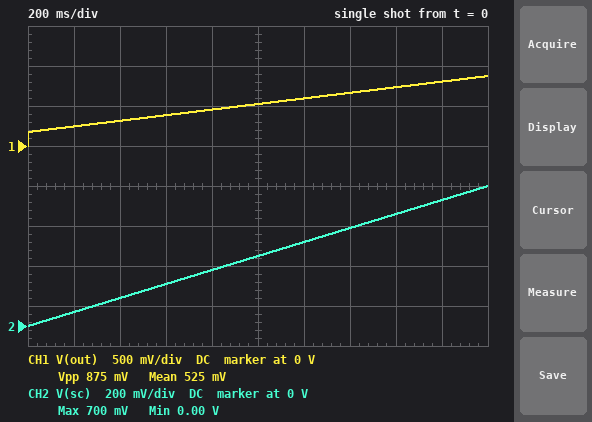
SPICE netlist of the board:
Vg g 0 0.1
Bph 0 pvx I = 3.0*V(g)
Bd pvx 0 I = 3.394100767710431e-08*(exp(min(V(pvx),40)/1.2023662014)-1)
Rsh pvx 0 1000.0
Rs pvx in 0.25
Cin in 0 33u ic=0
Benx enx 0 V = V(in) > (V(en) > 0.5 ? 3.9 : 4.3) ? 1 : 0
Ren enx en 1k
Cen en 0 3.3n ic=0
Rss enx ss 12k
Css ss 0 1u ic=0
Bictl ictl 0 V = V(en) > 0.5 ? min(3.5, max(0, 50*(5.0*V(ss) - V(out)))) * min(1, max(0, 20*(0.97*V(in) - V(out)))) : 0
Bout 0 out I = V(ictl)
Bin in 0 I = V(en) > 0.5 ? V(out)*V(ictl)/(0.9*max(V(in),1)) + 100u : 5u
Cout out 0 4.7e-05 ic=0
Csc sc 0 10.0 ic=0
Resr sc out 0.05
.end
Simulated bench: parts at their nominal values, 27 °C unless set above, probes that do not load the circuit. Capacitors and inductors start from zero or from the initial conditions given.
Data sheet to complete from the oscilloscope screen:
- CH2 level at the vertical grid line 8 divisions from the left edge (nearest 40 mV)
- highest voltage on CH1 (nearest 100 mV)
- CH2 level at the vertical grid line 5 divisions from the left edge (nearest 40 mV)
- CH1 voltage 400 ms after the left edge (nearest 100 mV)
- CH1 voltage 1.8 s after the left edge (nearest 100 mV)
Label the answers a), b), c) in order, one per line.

a) 560 mV
b) 900 mV
c) 360 mV
d) 300 mV
e) 800 mV
